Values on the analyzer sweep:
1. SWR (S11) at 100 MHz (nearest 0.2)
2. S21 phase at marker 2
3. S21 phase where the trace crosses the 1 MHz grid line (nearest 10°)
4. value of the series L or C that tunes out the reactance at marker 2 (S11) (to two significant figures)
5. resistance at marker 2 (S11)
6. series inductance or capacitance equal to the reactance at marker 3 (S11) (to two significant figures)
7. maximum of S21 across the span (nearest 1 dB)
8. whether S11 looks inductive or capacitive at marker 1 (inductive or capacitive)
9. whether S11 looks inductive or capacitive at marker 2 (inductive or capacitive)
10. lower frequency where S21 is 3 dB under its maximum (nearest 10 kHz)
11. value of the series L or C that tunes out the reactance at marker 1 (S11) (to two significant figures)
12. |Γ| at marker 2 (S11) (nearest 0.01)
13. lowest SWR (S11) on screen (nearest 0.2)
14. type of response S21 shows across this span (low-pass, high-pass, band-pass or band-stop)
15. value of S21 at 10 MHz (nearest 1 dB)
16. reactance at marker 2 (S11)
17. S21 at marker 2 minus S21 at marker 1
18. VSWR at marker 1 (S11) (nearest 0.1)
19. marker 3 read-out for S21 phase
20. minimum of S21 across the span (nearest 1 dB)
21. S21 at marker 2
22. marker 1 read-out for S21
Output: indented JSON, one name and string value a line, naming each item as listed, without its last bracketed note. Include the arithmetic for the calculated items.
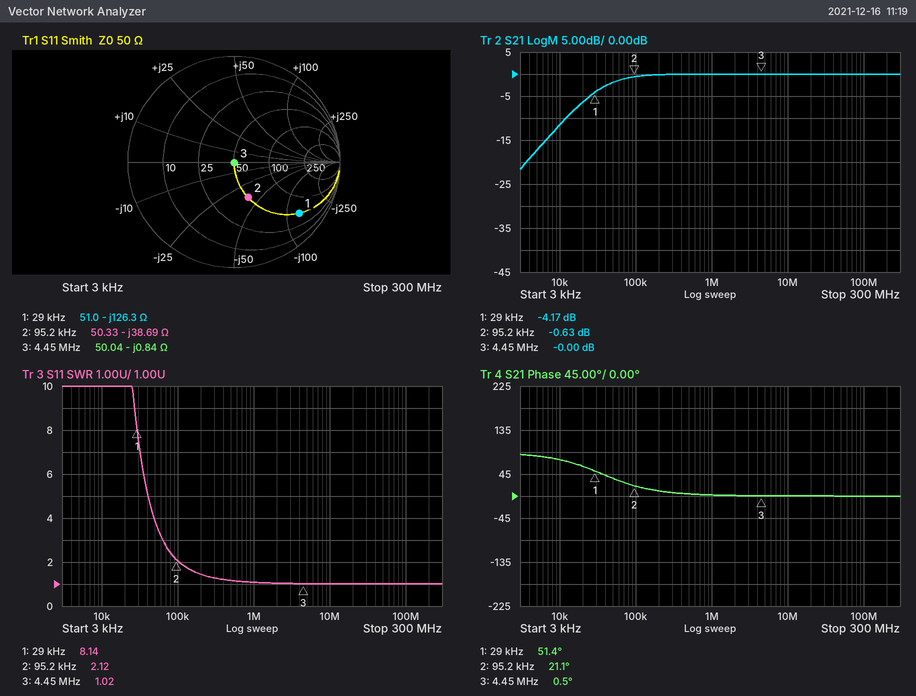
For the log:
{
  "SWR (S11) at 100 MHz": "1.0",
  "S21 phase at marker 2": "21.1°",
  "S21 phase where the trace crosses the 1 MHz grid line": "0°",
  "value of the series L or C that tunes out the reactance at marker 2 (S11)": "L = 38.69 Ω/(2π × 95.2 kHz) ≈ 65 µH",
  "resistance at marker 2": "50.33 Ω",
  "series inductance or capacitance equal to the reactance at marker 3 (S11)": "C = 1/(2π × 4.45 MHz × 0.84 Ω) ≈ 43 nF",
  "maximum of S21 across the span": "0 dB",
  "whether S11 looks inductive or capacitive at marker 1": "capacitive",
  "whether S11 looks inductive or capacitive at marker 2": "capacitive",
  "lower frequency where S21 is 3 dB under its maximum": "40 kHz",
  "value of the series L or C that tunes out the reactance at marker 1 (S11)": "L = 126.3 Ω/(2π × 29 kHz) ≈ 693 µH, so 690 µH to two significant figures",
  "|Γ| at marker 2 (S11)": "0.36",
  "lowest SWR (S11) on screen": "1.0",
  "type of response S21 shows across this span": "high-pass",
  "value of S21 at 10 MHz": "0 dB",
  "reactance at marker 2": "-38.69 Ω",
  "S21 at marker 2 minus S21 at marker 1": "-0.63 − (-4.17) = 3.54 dB",
  "VSWR at marker 1 (S11)": "8.1",
  "marker 3 read-out for S21 phase": "0.5°",
  "minimum of S21 across the span": "-22 dB",
  "S21 at marker 2": "-0.63 dB",
  "marker 1 read-out for S21": "-4.17 dB"
}
